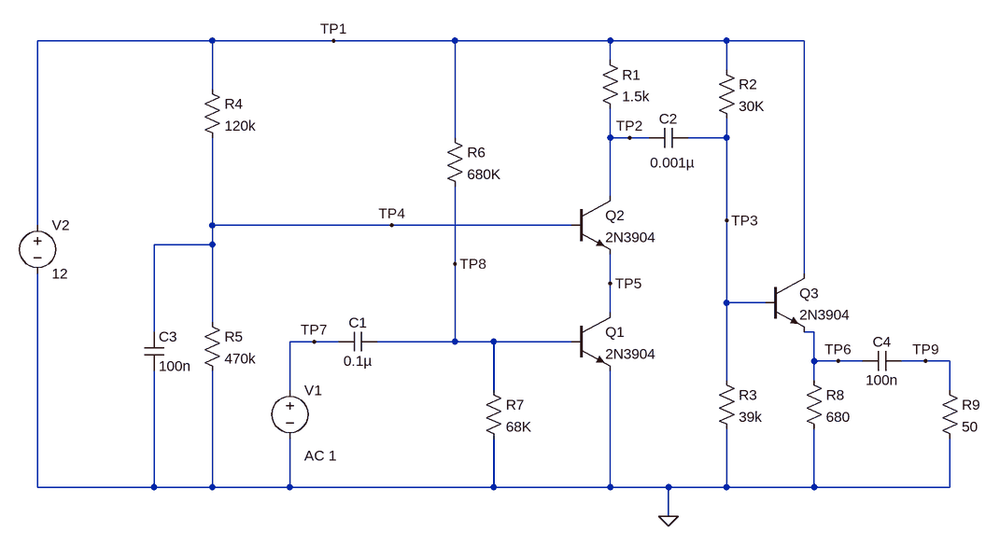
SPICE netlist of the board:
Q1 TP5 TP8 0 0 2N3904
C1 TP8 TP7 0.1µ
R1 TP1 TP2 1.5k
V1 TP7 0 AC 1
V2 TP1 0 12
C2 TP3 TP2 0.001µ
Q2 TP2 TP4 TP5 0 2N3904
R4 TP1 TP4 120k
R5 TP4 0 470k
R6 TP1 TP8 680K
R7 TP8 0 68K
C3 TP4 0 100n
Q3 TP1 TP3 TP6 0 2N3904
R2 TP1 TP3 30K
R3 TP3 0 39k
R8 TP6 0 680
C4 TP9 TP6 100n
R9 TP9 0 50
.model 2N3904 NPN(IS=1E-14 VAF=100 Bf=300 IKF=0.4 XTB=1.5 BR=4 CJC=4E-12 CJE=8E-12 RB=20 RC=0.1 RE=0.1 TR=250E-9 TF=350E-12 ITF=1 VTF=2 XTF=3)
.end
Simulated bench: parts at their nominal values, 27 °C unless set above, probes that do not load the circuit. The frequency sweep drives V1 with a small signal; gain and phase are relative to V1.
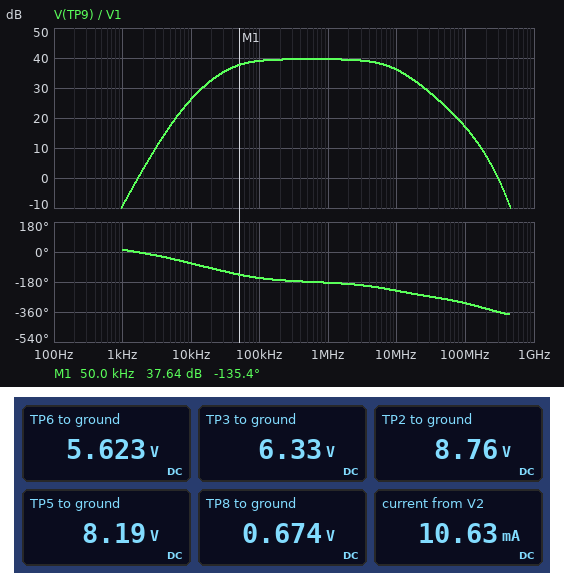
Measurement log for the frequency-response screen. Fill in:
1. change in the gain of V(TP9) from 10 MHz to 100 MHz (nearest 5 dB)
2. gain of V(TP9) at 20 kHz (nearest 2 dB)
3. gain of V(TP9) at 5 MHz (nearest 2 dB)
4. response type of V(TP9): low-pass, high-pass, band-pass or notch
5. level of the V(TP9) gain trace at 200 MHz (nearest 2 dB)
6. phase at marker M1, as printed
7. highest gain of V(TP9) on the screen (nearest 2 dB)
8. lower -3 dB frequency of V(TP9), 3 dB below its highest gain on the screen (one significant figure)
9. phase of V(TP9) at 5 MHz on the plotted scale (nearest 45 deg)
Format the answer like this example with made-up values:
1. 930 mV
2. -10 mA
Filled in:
1. -20 dB
2. 32 dB
3. 38 dB
4. band-pass
5. 8 dB
6. -135.4 deg
7. 40 dB
8. 40 kHz
9. -225 deg
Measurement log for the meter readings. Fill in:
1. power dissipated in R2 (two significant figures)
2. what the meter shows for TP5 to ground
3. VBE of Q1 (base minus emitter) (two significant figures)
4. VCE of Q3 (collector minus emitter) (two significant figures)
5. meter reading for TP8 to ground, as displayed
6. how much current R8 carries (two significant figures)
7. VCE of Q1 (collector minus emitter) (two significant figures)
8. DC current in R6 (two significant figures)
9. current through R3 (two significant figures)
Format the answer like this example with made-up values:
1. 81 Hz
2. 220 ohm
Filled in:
1. 1.1 mW
2. 8.19 V
3. 670 mV
4. 6.4 V
5. 0.674 V
6. 8.3 mA
7. 8.2 V
8. 17 µA
9. 160 µA
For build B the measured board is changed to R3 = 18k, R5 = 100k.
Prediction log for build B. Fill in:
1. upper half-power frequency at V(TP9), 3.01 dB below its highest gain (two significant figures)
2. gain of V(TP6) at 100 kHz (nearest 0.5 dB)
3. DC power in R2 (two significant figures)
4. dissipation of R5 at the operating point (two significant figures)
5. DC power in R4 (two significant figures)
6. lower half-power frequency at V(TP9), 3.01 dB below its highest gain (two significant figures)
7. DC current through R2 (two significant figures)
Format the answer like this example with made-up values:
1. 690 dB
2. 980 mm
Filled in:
1. 11 MHz
2. 38.5 dB
3. 2.0 mW
4. 260 µW
5. 400 µW
6. 39 kHz
7. 260 µA
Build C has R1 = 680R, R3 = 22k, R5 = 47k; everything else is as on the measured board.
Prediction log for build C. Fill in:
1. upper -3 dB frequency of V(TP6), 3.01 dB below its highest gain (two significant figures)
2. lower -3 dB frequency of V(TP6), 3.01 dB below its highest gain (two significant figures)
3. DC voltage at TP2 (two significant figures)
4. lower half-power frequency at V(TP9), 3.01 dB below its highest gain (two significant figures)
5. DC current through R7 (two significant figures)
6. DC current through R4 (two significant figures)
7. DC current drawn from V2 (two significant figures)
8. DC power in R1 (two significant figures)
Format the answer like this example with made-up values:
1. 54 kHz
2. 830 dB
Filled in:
1. 21 MHz
2. 14 kHz
3. 11 V
4. 41 kHz
5. 9.9 µA
6. 74 µA
7. 8.4 mA
8. 2.8 mW
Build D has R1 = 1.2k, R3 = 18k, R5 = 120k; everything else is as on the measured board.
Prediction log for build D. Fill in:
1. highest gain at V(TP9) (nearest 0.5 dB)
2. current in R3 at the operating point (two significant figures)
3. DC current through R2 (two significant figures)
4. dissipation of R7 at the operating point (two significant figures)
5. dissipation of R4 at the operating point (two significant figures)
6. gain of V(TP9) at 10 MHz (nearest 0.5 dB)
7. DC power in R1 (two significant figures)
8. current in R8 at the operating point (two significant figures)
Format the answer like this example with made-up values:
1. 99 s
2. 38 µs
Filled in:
1. 37.0 dB
2. 240 µA
3. 260 µA
4. 6.7 µW
5. 340 µW
6. 35.0 dB
7. 5.3 mW
8. 5.3 mA
